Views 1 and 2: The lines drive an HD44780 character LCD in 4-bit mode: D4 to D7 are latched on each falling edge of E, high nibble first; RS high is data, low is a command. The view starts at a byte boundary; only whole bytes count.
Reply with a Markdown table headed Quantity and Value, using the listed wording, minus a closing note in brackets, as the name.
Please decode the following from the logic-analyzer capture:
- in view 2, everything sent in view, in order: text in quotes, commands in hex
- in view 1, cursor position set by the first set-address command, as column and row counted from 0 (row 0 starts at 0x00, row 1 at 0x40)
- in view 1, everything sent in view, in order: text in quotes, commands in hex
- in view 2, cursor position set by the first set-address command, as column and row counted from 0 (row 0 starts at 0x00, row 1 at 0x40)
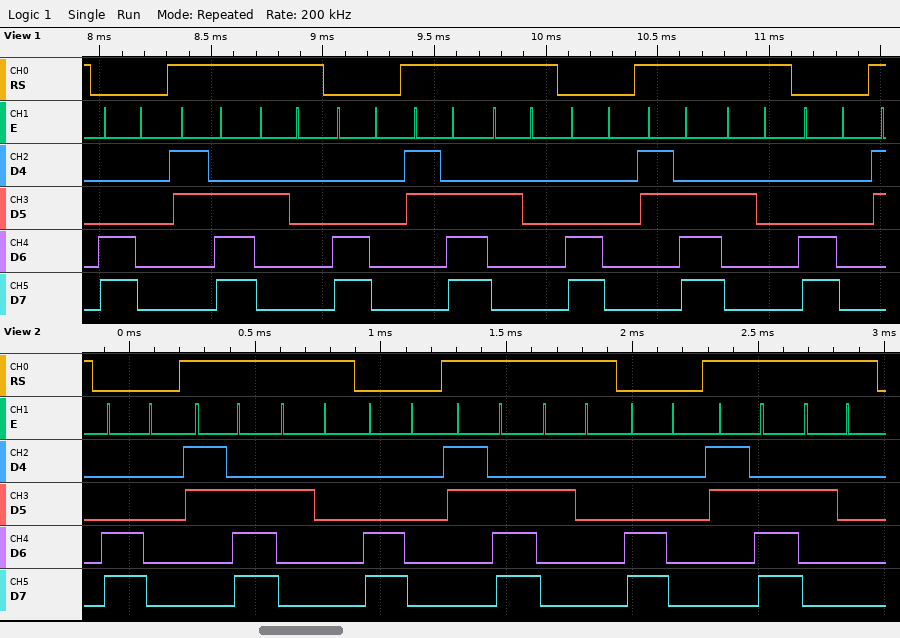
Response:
| Quantity | Value |
|---|---|
| in view 2, everything sent in view, in order: text in quotes, commands in hex | 0xC0 "> " 0xC0 "> " 0xC0 "> " |
| in view 1, cursor position set by the first set-address command, as column and row counted from 0 | column 0, row 1 |
| in view 1, everything sent in view, in order: text in quotes, commands in hex | 0xC0 "> " 0xC0 "> " 0xC0 "> " 0xC0 |
| in view 2, cursor position set by the first set-address command, as column and row counted from 0 | column 0, row 1 |
